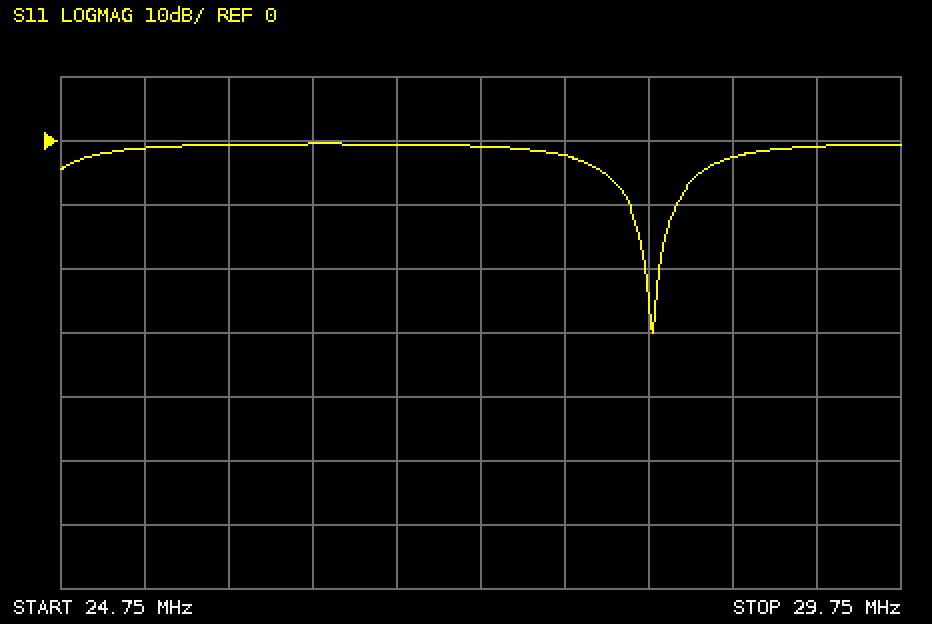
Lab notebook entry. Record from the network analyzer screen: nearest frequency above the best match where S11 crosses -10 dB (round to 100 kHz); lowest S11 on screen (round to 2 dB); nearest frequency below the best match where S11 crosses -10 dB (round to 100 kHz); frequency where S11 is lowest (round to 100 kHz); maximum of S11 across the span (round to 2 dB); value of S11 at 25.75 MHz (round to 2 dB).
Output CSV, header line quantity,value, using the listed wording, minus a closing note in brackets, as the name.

quantity,value
nearest frequency above the best match where S11 crosses -10 dB,28.4 MHz
lowest S11 on screen,-30 dB
nearest frequency below the best match where S11 crosses -10 dB,28.1 MHz
frequency where S11 is lowest,28.3 MHz
maximum of S11 across the span,0 dB
value of S11 at 25.75 MHz,0 dB
